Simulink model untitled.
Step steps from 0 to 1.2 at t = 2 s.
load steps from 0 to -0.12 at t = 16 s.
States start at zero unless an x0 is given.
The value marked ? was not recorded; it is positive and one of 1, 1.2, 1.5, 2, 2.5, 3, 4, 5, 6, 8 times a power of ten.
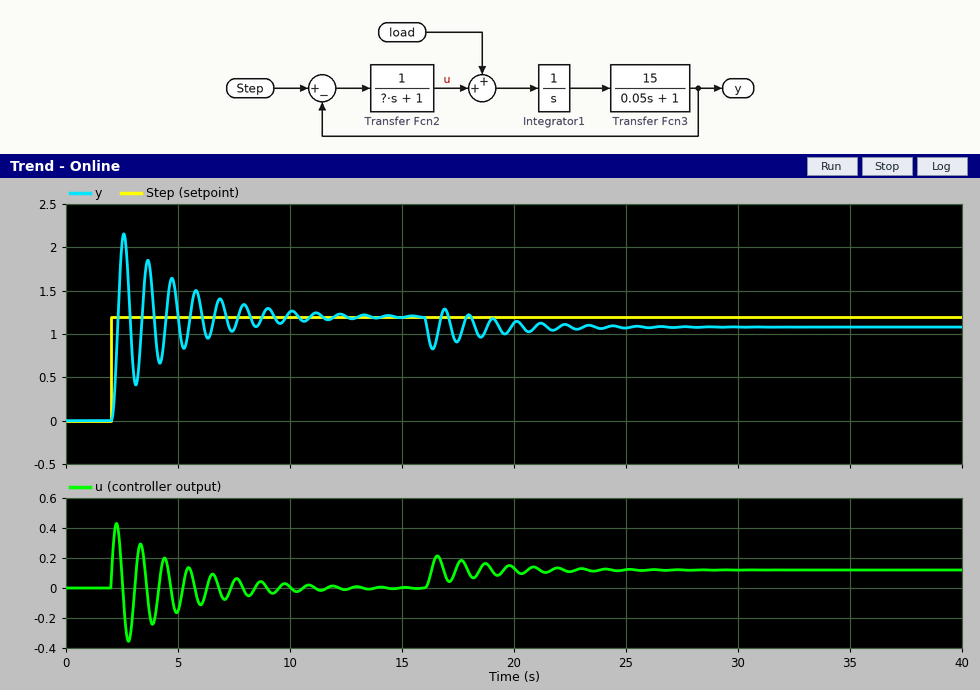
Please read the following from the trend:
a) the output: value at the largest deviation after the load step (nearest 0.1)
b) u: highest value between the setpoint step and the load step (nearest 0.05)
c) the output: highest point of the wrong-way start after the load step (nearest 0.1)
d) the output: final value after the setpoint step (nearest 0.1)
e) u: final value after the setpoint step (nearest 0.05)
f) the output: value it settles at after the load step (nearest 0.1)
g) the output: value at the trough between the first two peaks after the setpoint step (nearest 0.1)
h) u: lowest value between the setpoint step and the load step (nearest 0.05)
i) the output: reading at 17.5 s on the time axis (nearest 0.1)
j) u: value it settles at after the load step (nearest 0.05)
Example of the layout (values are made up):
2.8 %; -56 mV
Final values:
0.8; 0.45; 1.3; 1.2; 0.00; 1.1; 0.4; -0.35; 0.9; 0.10
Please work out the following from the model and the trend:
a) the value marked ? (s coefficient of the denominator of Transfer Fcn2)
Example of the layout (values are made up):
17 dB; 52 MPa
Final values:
0.4
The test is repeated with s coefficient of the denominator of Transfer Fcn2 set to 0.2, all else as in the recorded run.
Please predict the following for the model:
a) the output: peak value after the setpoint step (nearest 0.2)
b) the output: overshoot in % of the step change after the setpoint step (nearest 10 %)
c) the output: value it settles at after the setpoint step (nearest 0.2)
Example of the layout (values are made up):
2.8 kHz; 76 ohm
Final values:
2.0; 70 %; 1.2
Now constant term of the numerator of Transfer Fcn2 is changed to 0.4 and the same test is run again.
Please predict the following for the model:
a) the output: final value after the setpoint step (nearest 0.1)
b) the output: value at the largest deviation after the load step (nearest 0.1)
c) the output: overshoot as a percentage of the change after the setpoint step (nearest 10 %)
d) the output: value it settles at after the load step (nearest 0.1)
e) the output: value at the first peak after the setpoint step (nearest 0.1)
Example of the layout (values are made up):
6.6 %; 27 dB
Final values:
1.2; 0.6; 50 %; 0.9; 1.8
